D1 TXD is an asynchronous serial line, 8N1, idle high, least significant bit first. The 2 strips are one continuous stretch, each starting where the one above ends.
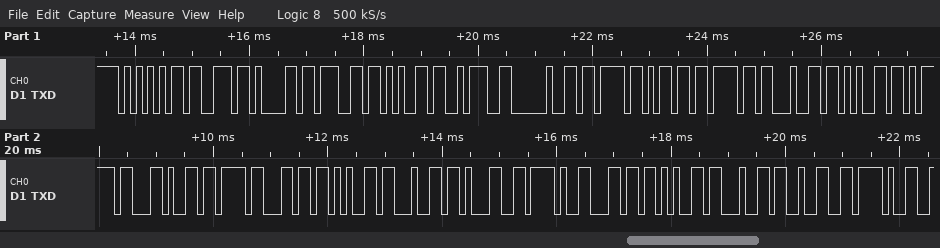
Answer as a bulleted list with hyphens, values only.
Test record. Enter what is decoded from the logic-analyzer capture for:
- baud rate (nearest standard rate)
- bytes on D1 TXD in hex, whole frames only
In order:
- 9600 baud
- 55 73 61 67 65 3A 20 7B 6D 6F 64 65 7D 2C 7B 6C 65 64 31 2F 6C 65 64 32 2F
